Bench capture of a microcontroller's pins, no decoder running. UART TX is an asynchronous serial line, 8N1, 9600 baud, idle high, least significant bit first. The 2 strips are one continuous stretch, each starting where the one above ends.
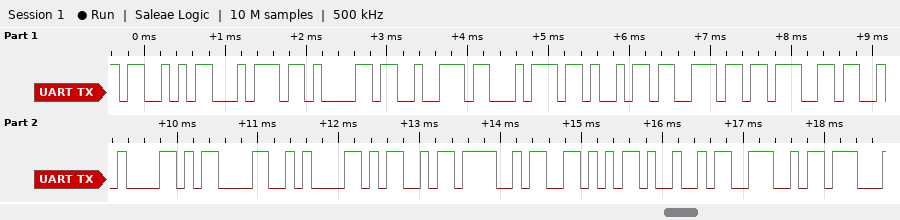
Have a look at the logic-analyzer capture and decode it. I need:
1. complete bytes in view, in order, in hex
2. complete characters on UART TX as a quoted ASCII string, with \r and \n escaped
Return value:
53 74 61 72 74 69 6E 67 0A 0D 0A 4D 4F 56 49 4E
"Starting\n\r\nMOVIN"
